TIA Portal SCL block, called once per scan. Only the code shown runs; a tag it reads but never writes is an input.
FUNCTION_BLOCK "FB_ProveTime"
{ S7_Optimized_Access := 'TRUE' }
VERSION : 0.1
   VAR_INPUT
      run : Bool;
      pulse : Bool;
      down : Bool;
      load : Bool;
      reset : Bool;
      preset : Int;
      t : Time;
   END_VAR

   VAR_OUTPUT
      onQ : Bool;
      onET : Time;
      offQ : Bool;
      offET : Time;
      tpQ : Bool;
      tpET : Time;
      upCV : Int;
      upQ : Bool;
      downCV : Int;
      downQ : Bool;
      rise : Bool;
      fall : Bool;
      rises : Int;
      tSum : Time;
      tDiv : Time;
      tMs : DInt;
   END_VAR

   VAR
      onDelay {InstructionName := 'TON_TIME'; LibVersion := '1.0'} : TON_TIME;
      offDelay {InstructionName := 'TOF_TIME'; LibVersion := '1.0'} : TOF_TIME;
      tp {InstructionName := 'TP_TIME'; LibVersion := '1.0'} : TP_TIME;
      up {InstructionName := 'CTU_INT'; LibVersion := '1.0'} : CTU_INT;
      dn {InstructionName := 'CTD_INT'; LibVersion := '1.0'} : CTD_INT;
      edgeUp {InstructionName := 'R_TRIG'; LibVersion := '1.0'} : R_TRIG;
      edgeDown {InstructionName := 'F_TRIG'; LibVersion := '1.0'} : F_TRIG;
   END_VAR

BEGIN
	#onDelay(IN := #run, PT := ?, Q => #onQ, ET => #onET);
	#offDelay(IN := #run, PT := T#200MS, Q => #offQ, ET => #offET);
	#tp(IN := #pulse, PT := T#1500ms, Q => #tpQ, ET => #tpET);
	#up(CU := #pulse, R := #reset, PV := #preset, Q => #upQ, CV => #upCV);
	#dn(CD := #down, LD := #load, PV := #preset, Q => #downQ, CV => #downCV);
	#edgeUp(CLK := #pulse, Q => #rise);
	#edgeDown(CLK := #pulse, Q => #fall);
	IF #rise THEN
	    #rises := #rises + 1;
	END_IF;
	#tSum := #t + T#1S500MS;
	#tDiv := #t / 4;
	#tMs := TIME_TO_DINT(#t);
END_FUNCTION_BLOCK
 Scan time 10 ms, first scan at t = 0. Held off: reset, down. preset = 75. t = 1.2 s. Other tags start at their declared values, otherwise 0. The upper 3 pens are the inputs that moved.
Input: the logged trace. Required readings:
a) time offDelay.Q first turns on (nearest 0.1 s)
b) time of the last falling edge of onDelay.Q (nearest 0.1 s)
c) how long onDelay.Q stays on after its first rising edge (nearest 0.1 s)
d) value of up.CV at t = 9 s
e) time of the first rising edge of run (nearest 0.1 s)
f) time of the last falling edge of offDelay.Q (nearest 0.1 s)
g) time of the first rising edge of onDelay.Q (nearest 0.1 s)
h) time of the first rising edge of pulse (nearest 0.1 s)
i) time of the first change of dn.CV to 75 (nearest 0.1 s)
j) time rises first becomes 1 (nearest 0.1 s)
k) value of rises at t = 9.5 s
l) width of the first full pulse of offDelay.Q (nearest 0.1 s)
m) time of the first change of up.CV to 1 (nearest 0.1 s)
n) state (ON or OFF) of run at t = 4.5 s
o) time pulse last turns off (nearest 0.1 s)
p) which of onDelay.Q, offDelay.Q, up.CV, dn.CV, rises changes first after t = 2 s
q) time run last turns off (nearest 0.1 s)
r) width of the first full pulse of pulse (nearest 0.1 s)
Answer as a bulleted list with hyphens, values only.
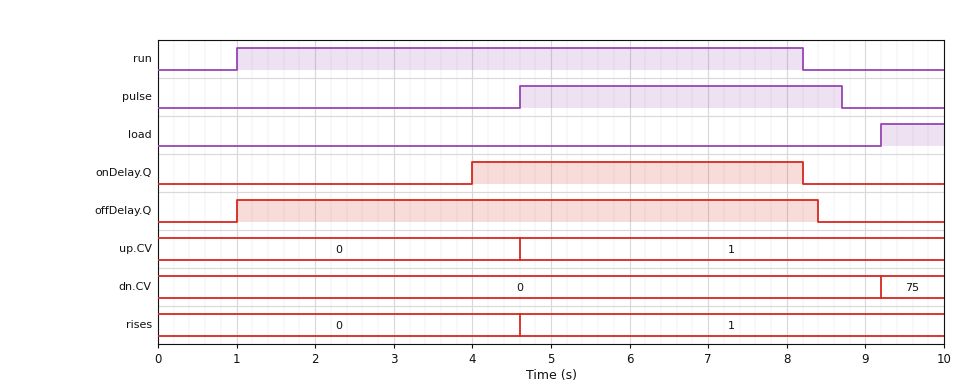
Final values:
- 1.0 s
- 8.2 s
- 4.2 s
- 1
- 1.0 s
- 8.4 s
- 4.0 s
- 4.6 s
- 9.2 s
- 4.6 s
- 1
- 7.4 s
- 4.6 s
- ON
- 8.7 s
- onDelay.Q
- 8.2 s
- 4.1 s
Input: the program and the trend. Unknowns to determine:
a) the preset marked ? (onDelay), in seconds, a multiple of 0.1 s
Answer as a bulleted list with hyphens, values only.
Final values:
- 3.0 s
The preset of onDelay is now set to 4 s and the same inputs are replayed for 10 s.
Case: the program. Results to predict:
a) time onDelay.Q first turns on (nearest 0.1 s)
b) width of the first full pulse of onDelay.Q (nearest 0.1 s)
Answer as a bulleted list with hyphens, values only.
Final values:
- 5.0 s
- 3.2 s
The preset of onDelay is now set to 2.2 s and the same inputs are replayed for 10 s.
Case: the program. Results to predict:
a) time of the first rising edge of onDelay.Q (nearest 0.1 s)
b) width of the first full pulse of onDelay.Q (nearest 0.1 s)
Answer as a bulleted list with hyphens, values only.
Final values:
- 3.2 s
- 5.0 s
